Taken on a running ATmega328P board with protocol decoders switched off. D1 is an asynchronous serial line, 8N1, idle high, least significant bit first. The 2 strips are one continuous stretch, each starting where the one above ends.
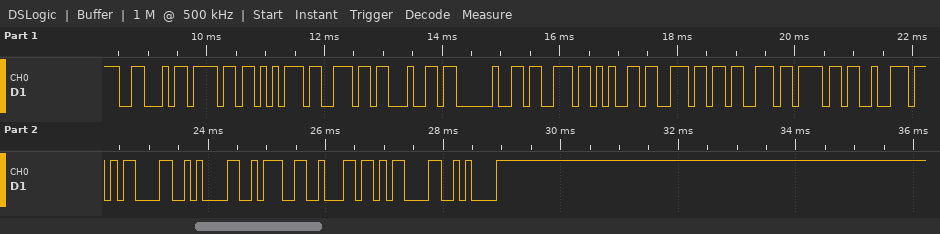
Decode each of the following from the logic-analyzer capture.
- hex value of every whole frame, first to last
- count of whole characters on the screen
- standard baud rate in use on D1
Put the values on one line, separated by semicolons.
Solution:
46 6F 75 6E 64 20 73 65 6E 73 6F 72 0D 0A 3A 62 0D 0A; 18; 9600 baud
